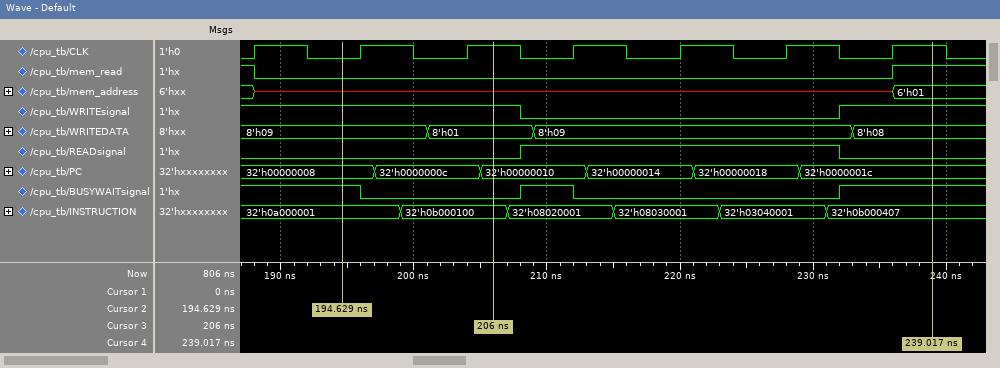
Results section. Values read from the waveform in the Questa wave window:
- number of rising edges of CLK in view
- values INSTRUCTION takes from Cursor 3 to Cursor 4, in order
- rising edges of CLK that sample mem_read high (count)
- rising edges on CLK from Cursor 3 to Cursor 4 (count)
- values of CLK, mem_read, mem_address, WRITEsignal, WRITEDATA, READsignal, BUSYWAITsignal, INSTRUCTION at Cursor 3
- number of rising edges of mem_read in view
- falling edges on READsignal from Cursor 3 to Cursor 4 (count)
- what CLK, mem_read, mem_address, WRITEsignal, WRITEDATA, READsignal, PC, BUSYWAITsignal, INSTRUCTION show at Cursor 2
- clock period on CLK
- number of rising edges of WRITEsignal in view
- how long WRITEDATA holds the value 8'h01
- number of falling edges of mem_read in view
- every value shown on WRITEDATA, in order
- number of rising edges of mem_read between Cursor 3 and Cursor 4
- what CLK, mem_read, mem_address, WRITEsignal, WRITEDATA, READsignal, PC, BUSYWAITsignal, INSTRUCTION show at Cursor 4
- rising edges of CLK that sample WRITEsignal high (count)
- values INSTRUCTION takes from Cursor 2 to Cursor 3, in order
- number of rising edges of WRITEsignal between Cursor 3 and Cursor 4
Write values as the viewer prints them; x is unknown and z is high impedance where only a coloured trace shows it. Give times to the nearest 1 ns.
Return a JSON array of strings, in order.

["7", "32'h0b000100, 32'h08020001, 32'h08030001, 32'h03040001, 32'h0b000407", "1", "4", "CLK=1, mem_read=0, mem_address=x, WRITEsignal=1, WRITEDATA=8'h01, READsignal=0, BUSYWAITsignal=0, INSTRUCTION=32'h0b000100", "1", "1", "CLK=0, mem_read=0, mem_address=x, WRITEsignal=1, WRITEDATA=8'h09, READsignal=0, PC=32'h00000008, BUSYWAITsignal=1, INSTRUCTION=32'h0a000001", "8 ns", "1", "8 ns", "1", "8'h09, 8'h01, 8'h09, 8'h08", "1", "CLK=1, mem_read=1, mem_address=6'h01, WRITEsignal=1, WRITEDATA=8'h08, READsignal=0, PC=32'h0000001c, BUSYWAITsignal=1, INSTRUCTION=32'h0b000407", "4", "32'h0a000001, 32'h0b000100", "1"]
